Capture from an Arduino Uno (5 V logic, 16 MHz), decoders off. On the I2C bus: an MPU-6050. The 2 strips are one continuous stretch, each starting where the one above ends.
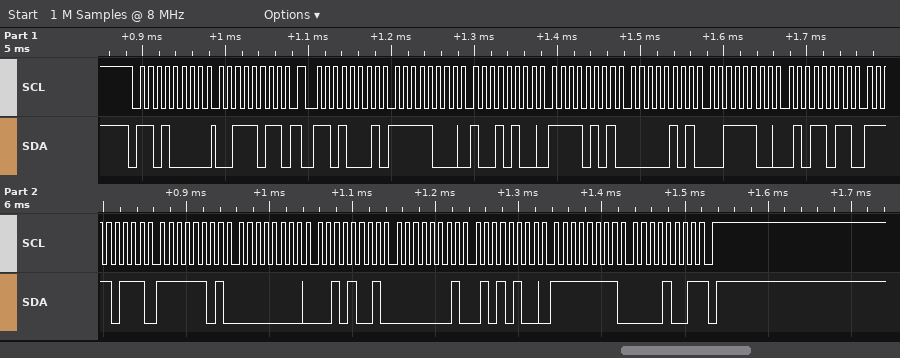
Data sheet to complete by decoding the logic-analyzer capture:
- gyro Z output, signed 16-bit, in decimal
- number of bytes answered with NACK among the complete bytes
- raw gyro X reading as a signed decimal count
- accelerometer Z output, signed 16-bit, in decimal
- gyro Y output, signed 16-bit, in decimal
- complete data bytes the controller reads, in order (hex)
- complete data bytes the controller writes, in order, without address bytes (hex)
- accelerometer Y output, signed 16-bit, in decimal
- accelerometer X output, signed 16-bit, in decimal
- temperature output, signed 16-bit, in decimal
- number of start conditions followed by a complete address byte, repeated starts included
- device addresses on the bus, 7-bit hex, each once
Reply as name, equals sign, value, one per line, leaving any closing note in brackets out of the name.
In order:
gyro Z output, signed 16-bit, in decimal = -247
number of bytes answered with NACK among the complete bytes = 1
raw gyro X reading as a signed decimal count = 41
accelerometer Z output, signed 16-bit, in decimal = 15451
gyro Y output, signed 16-bit, in decimal = 340
complete data bytes the controller reads, in order = F8 94 F5 05 3C 5B F7 FD 00 29 01 54 FF 09
complete data bytes the controller writes, in order, without address bytes = 3B
accelerometer Y output, signed 16-bit, in decimal = -2811
accelerometer X output, signed 16-bit, in decimal = -1900
temperature output, signed 16-bit, in decimal = -2051
number of start conditions followed by a complete address byte, repeated starts included = 2
device addresses on the bus, 7-bit hex, each once = 0x68
